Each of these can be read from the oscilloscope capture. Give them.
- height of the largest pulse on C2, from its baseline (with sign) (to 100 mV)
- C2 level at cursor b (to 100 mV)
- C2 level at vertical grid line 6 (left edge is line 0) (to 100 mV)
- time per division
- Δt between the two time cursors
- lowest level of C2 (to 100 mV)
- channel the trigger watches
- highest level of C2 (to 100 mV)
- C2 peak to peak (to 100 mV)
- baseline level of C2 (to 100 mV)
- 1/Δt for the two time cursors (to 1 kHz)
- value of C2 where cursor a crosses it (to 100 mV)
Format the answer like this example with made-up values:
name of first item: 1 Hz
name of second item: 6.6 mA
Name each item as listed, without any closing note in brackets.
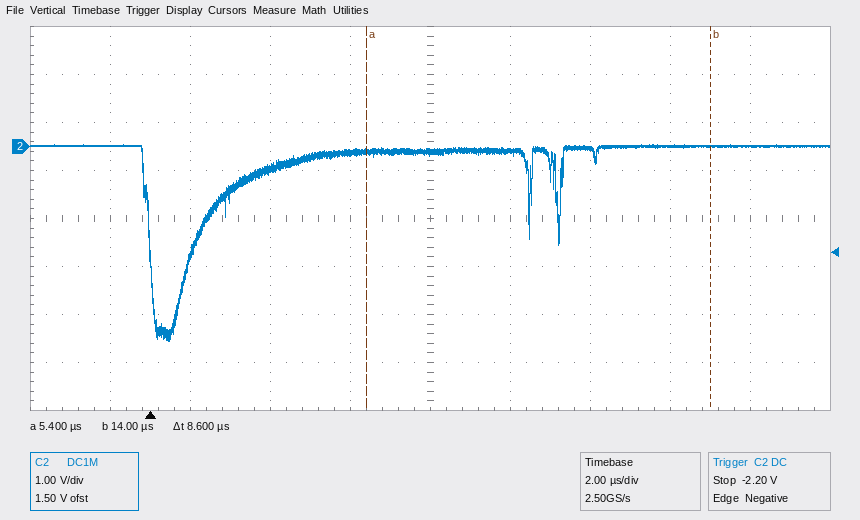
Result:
height of the largest pulse on C2, from its baseline (with sign): -4.1 V
C2 level at cursor b: 0.0 V
C2 level at vertical grid line 6 (left edge is line 0): -100 mV
time per division: 2 µs
Δt between the two time cursors: 8.6 µs
lowest level of C2: -4.1 V
channel the trigger watches: C2
highest level of C2: 0.0 V
C2 peak to peak: 4.1 V
baseline level of C2: 0.0 V
1/Δt for the two time cursors: 116 kHz
value of C2 where cursor a crosses it: -100 mV
